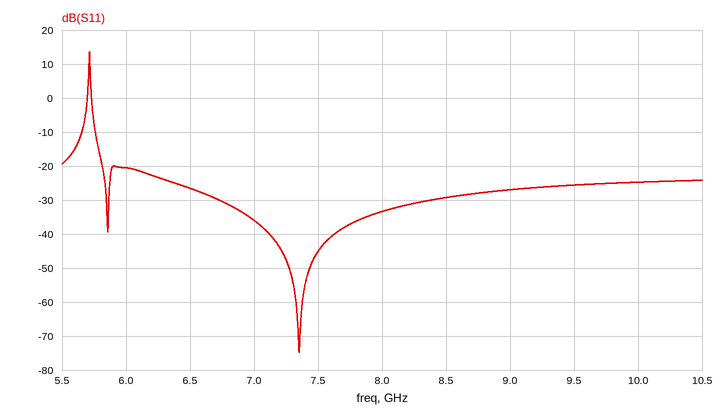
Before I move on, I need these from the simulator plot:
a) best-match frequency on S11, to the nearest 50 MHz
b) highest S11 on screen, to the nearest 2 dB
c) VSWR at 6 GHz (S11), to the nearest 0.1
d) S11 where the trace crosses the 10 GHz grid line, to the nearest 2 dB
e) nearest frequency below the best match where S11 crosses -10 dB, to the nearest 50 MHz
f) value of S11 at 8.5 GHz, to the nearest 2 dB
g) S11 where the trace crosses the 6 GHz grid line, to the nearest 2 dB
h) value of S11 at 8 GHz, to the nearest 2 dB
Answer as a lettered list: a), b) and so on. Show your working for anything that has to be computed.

a) 7.35 GHz
b) 14 dB
c) |Γ| = 10^(-20/20) = 0.1000; VSWR = (1 + 0.1000)/(1 − 0.1000) ≈ 1.2
d) -24 dB
e) 5.75 GHz
f) -30 dB
g) -20 dB
h) -34 dB
